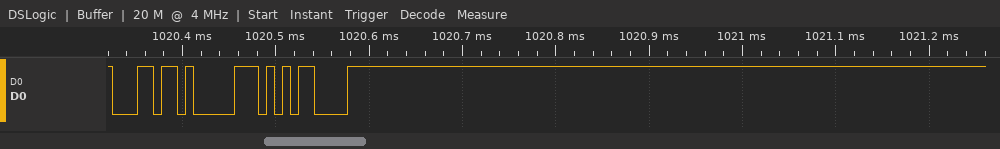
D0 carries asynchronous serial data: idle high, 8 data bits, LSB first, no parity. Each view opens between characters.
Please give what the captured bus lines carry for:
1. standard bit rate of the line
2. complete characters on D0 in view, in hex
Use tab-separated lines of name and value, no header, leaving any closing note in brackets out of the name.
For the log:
standard bit rate of the line	115200 baud
complete characters on D0 in view, in hex	6C, 70, 0D
